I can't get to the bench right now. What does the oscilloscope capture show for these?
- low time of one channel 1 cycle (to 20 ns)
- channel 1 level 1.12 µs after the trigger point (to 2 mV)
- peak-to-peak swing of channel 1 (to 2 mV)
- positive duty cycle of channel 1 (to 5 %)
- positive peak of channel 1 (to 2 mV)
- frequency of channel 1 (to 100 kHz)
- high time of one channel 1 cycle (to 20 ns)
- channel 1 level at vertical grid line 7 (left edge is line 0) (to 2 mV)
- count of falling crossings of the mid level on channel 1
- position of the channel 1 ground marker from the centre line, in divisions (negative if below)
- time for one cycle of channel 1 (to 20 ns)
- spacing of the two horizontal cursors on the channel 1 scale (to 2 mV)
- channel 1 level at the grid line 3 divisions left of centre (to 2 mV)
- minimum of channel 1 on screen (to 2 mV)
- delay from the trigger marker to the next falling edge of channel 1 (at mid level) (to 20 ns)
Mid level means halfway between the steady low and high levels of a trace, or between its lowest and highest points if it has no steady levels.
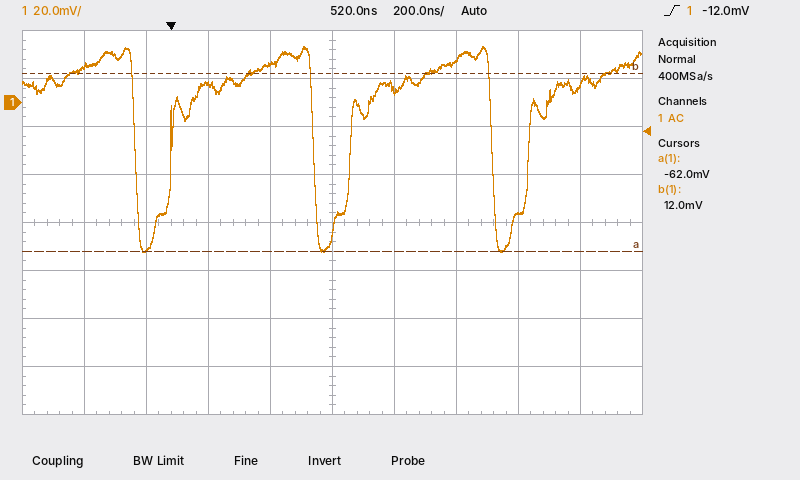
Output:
120 ns
-46 mV
86 mV
80 %
24 mV
1.7 MHz
460 ns
18 mV
3
+2.5 div
580 ns
74 mV
-62 mV
-62 mV
460 ns
